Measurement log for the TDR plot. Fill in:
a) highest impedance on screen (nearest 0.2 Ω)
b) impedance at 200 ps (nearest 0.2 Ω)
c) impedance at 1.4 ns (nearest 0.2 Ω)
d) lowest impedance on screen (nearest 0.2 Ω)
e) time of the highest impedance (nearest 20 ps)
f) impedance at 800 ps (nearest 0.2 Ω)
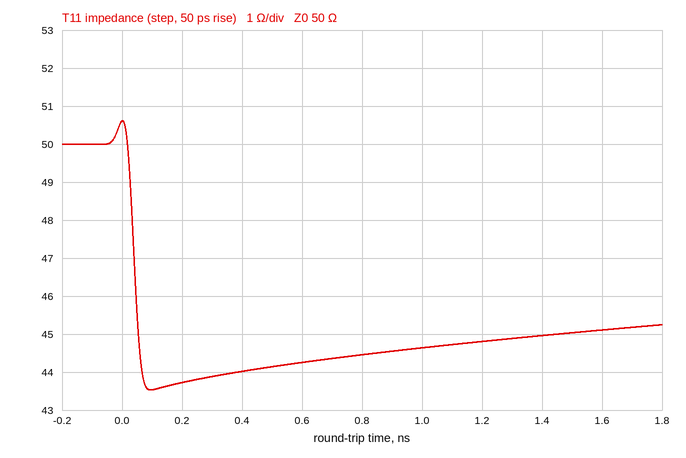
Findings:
50.6 Ω
43.8 Ω
45.0 Ω
43.6 Ω
0 ps
44.4 Ω
